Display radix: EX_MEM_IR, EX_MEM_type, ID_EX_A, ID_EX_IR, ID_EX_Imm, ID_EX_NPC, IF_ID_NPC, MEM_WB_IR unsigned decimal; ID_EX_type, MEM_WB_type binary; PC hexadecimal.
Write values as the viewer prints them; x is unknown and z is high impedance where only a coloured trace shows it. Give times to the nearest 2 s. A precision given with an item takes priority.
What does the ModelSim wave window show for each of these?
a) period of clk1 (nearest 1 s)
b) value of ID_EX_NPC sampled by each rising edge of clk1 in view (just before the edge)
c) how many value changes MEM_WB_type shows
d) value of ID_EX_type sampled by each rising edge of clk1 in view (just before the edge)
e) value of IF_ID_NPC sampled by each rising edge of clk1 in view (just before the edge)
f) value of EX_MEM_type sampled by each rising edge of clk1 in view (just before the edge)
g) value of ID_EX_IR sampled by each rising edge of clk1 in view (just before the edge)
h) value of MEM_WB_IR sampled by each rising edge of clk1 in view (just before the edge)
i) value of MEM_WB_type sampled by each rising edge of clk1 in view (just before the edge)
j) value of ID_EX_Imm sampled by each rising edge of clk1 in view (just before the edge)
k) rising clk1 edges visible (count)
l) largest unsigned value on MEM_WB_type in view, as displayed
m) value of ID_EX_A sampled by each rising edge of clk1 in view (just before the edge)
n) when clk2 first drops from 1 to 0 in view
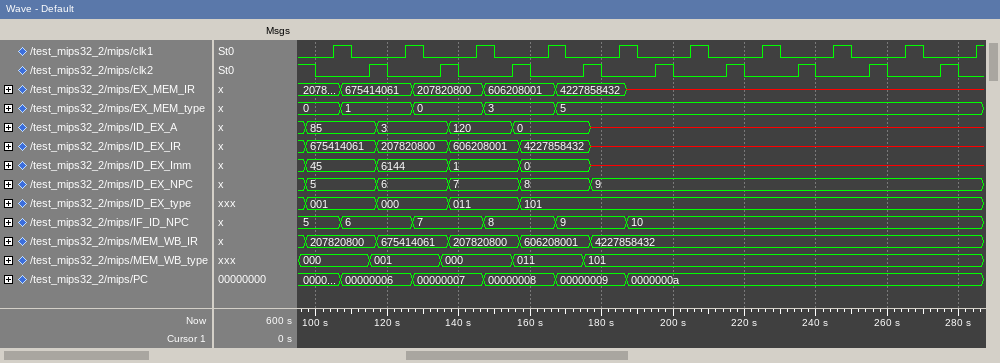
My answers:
20 s
5, 6, 7, 8, 9, 9, 9, 9, 9, 9
4
001, 000, 011, 101, 101, 101, 101, 101, 101, 101
5, 6, 7, 8, 9, 10, 10, 10, 10, 10
0, 1, 0, 3, 5, 5, 5, 5, 5, 5
675414061, 207820800, 606208001, 4227858432, x, x, x, x, x, x
207820800, 675414061, 207820800, 606208001, 4227858432, 4227858432, 4227858432, 4227858432, 4227858432, 4227858432
000, 001, 000, 011, 101, 101, 101, 101, 101, 101
45, 6144, 1, 0, x, x, x, x, x, x
10
101
85, 3, 120, 0, x, x, x, x, x, x
100 s
